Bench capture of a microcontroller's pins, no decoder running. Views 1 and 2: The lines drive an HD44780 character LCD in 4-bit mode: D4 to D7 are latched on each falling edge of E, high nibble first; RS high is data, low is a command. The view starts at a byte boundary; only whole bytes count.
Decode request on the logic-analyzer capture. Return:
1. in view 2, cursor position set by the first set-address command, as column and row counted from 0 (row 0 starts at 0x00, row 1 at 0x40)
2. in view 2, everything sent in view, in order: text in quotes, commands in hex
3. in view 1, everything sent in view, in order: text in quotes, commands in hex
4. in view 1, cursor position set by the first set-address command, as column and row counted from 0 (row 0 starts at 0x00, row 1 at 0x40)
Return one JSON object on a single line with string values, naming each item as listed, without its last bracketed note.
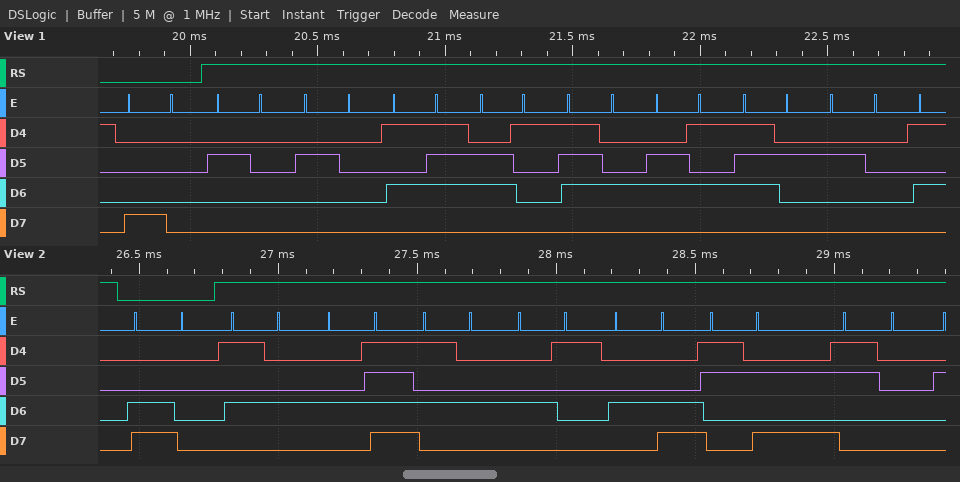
{"in view 2, cursor position set by the first set-address command, as column and row counted from 0": "column 0, row 1", "in view 2, everything sent in view, in order: text in quotes, commands in hex": "0xC0 \"TOTAL:0\"", "in view 1, everything sent in view, in order: text in quotes, commands in hex": "0x80 \"  Water \"", "in view 1, cursor position set by the first set-address command, as column and row counted from 0": "column 0, row 0"}
